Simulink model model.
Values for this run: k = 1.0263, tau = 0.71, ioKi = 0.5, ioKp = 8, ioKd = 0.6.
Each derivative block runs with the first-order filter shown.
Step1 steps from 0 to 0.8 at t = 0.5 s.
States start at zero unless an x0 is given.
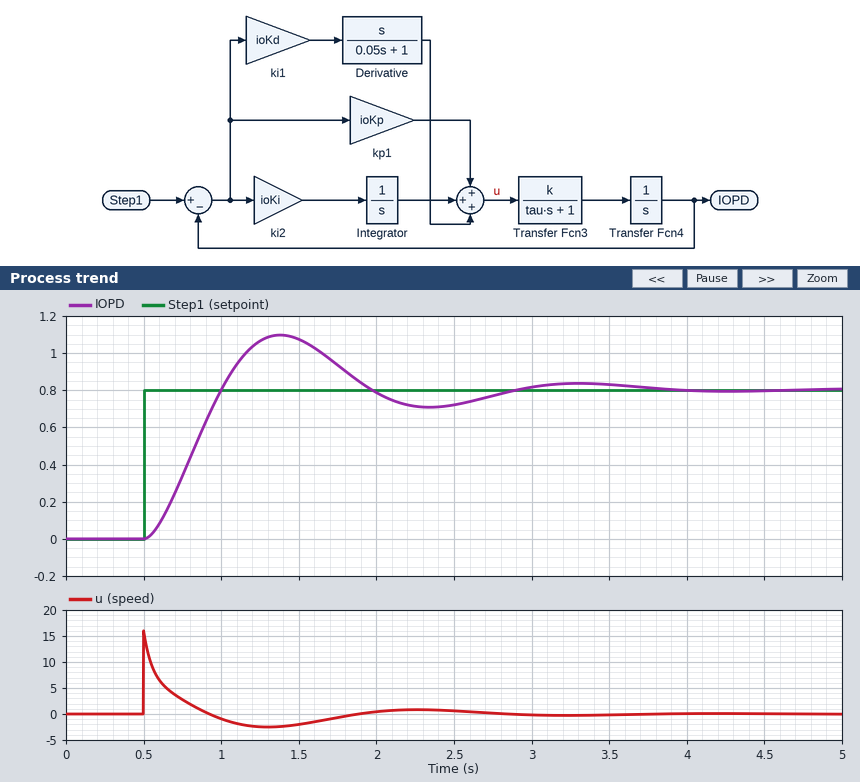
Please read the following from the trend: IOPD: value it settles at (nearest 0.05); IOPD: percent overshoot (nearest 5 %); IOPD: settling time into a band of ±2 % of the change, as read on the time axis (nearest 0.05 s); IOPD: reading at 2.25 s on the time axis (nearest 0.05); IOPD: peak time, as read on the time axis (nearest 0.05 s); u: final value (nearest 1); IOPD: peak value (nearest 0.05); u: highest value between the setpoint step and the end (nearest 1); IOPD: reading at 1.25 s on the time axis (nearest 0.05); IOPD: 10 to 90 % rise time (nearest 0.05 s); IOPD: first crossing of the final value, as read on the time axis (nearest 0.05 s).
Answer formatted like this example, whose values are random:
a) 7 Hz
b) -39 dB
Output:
a) 0.80
b) 35 %
c) 3.70 s
d) 0.70
e) 1.40 s
f) 0
g) 1.10
h) 16
i) 1.05
j) 0.35 s
k) 1.00 s
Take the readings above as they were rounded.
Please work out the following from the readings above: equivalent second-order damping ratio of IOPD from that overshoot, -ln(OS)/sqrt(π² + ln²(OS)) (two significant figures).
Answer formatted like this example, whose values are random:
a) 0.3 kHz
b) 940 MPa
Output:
a) 0.32
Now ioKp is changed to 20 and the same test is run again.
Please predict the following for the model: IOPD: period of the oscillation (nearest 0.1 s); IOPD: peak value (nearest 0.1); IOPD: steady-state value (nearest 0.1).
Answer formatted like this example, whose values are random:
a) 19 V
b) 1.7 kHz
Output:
a) 1.2 s
b) 1.2
c) 0.8
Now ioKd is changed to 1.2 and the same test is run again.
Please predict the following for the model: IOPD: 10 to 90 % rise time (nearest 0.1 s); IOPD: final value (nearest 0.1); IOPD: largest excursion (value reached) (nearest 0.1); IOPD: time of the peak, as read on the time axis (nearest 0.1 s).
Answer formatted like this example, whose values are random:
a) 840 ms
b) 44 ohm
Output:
a) 0.3 s
b) 0.8
c) 1.0
d) 1.3 s
